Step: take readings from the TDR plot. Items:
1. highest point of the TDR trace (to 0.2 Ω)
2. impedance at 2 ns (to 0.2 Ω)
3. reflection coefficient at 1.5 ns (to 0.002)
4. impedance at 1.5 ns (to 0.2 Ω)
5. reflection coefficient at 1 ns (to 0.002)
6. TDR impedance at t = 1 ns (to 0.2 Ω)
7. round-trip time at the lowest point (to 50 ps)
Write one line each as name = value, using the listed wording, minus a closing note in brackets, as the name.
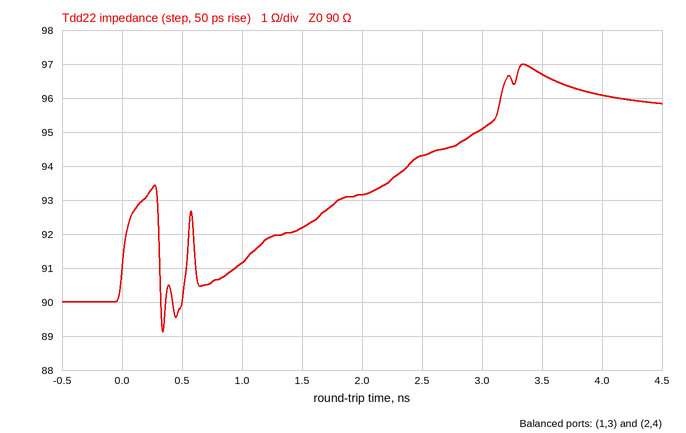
highest point of the TDR trace = 97.0 Ω
impedance at 2 ns = 93.2 Ω
reflection coefficient at 1.5 ns = +0.012
impedance at 1.5 ns = 92.2 Ω
reflection coefficient at 1 ns = +0.006
TDR impedance at t = 1 ns = 91.2 Ω
round-trip time at the lowest point = 350 ps
